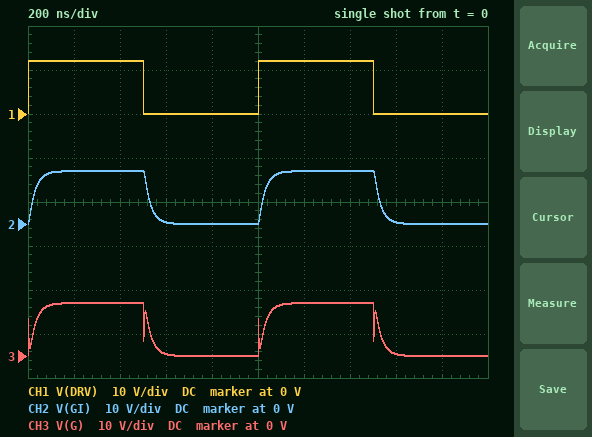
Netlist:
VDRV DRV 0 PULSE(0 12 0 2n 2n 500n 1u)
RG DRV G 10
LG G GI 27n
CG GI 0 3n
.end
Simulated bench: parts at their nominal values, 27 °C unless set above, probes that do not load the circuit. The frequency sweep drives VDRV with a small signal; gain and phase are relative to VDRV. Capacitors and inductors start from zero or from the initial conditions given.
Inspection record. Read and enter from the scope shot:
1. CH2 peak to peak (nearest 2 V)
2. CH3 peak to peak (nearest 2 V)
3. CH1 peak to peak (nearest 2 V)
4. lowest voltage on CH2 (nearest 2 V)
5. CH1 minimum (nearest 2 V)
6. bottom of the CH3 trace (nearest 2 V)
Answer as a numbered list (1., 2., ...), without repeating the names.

1. 12 V
2. 12 V
3. 12 V
4. 0 V
5. 0 V
6. 0 V
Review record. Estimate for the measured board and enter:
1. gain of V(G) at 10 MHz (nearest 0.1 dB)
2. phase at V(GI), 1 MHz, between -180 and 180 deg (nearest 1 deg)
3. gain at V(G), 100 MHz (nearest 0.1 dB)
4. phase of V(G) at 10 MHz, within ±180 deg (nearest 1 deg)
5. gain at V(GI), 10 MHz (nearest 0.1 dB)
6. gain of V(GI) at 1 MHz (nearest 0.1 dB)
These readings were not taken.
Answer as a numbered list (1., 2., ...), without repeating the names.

1. -9.4 dB
2. -11 deg
3. -1.4 dB
4. -70 deg
5. -6.0 dB
6. -0.1 dB
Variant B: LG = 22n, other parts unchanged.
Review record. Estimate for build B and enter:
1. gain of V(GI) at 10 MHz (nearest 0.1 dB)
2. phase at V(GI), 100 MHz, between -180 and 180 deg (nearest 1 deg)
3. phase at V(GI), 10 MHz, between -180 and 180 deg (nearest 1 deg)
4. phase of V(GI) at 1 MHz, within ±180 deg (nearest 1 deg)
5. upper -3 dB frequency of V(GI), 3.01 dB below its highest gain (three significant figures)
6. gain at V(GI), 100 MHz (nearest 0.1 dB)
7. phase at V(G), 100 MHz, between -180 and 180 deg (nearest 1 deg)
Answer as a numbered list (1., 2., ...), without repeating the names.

1. -6.1 dB
2. -143 deg
3. -69 deg
4. -11 deg
5. 5.72 MHz
6. -29.9 dB
7. 37 deg
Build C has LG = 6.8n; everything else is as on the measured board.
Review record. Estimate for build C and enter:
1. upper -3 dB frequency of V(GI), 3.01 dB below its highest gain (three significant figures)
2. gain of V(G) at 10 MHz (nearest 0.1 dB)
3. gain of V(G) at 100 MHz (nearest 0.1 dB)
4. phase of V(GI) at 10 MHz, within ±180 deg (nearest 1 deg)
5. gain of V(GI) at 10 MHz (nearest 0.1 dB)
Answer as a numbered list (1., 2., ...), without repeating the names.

1. 5.43 MHz
2. -7.2 dB
3. -9.1 dB
4. -64 deg
5. -6.4 dB
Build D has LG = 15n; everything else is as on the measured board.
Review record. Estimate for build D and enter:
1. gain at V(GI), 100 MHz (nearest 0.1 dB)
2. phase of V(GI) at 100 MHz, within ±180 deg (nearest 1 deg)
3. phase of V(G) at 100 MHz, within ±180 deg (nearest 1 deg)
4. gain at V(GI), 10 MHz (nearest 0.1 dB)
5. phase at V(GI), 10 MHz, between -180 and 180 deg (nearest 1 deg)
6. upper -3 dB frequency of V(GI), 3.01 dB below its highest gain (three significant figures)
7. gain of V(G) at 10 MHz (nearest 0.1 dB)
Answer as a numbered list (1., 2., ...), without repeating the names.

1. -28.0 dB
2. -132 deg
3. 48 deg
4. -6.3 dB
5. -66 deg
6. 5.58 MHz
7. -8.0 dB
